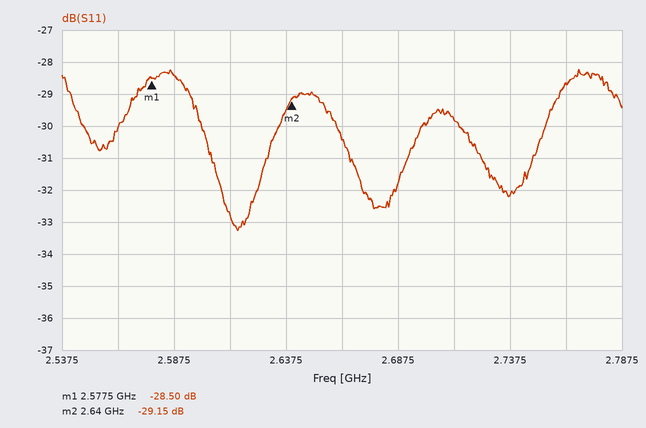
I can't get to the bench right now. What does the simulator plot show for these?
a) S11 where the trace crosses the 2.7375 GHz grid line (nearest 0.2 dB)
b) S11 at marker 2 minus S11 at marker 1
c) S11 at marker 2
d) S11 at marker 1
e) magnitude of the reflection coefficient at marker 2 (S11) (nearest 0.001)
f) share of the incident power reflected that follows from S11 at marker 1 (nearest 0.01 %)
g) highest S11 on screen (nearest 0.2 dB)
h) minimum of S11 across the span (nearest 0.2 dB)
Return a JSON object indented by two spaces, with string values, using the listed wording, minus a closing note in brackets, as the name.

{
  "S11 where the trace crosses the 2.7375 GHz grid line": "-32.2 dB",
  "S11 at marker 2 minus S11 at marker 1": "-0.65 dB",
  "S11 at marker 2": "-29.15 dB",
  "S11 at marker 1": "-28.50 dB",
  "magnitude of the reflection coefficient at marker 2 (S11)": "0.035",
  "share of the incident power reflected that follows from S11 at marker 1": "0.14 %",
  "highest S11 on screen": "-28.2 dB",
  "minimum of S11 across the span": "-33.2 dB"
}
